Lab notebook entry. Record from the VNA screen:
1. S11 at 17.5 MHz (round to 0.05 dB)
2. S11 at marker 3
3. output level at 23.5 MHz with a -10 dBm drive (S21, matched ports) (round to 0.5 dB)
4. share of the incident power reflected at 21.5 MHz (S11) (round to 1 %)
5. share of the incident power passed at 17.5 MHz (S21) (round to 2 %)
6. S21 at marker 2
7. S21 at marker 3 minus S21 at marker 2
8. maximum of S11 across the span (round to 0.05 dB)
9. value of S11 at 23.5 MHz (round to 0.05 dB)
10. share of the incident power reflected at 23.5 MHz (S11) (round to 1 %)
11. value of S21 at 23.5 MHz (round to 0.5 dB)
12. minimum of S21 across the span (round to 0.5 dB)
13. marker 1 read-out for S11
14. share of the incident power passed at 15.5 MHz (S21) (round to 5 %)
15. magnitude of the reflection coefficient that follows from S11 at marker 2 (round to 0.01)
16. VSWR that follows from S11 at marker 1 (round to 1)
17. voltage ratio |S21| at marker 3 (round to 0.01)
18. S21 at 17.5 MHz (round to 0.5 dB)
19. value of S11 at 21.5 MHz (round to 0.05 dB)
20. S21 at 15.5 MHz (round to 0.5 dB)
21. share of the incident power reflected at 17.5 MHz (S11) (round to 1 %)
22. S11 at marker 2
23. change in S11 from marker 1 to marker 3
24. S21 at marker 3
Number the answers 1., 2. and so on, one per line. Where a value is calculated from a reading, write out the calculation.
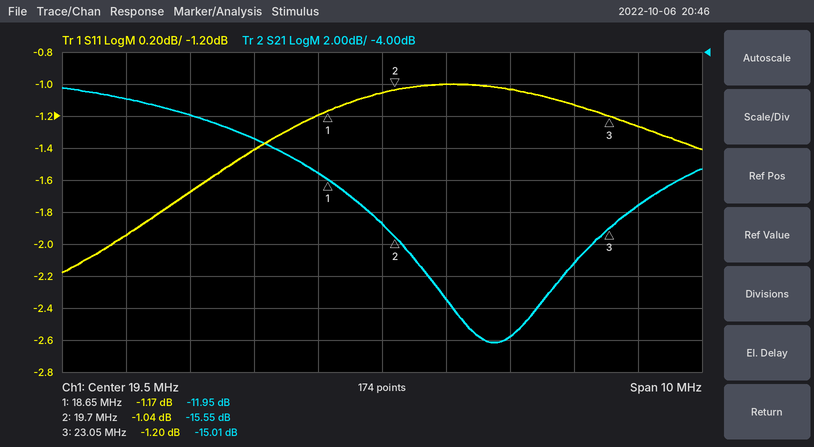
1. -1.40 dB
2. -1.20 dB
3. -10 dBm + (-13.5 dB) = -23.5 dBm
4. 10^(-1.05/10) ≈ 79 %
5. 10^(-9.5/10) ≈ 11.2 %, so 12 % to the nearest 2 %
6. -15.55 dB
7. -15.01 − (-15.55) = 0.54 dB
8. -1.00 dB
9. -1.25 dB
10. 10^(-1.25/10) ≈ 75 %
11. -13.5 dB
12. -22.0 dB
13. -1.17 dB
14. 10^(-7/10) ≈ 20 %
15. 10^(-1.04/20) ≈ 0.89
16. (1 + 0.8740)/(1 − 0.8740) ≈ 15
17. 10^(-15.01/20) ≈ 0.18
18. -9.5 dB
19. -1.05 dB
20. -7.0 dB
21. 10^(-1.4/10) ≈ 72 %
22. -1.04 dB
23. -1.2 − (-1.17) = -0.03 dB
24. -15.01 dB
